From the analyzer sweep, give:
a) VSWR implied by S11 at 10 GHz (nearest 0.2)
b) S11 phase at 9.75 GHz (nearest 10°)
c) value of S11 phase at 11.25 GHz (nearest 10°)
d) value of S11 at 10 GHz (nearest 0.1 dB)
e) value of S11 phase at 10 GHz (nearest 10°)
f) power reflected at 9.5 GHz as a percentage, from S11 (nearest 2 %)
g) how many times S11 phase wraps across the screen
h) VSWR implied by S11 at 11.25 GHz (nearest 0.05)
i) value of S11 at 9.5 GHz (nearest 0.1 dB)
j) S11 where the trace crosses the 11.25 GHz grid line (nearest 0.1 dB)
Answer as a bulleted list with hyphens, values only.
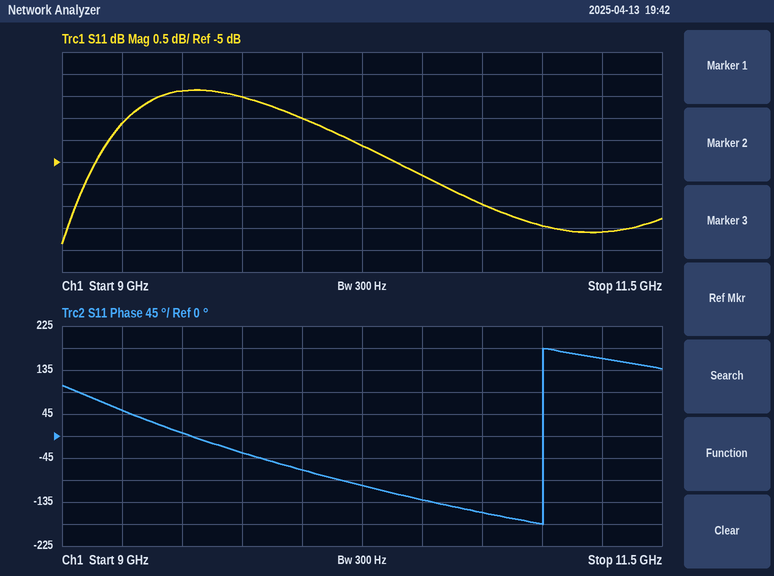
- 4.4
- -30°
- 160°
- -4.0 dB
- -70°
- 46 %
- 1
- 2.75
- -3.4 dB
- -6.6 dB
